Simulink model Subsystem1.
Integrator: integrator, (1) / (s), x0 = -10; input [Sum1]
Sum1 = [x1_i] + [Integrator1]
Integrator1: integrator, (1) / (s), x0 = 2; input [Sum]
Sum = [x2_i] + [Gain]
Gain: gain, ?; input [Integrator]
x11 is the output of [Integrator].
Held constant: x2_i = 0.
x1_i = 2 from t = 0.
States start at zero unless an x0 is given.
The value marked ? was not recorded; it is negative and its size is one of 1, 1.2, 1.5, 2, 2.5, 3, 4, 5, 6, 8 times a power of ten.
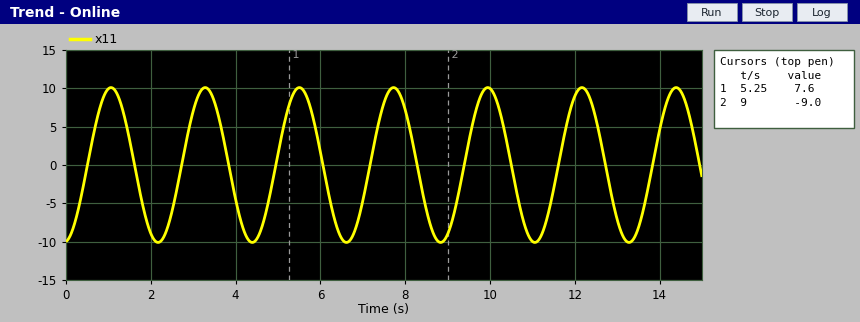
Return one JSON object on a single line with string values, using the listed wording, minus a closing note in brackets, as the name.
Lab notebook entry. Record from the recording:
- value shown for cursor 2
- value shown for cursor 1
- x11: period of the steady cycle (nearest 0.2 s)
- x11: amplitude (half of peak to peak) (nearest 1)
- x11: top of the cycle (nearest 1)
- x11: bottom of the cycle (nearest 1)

{"value shown for cursor 2": "-9.0", "value shown for cursor 1": "7.6", "x11: period of the steady cycle": "2.2 s", "x11: amplitude (half of peak to peak)": "10", "x11: top of the cycle": "10", "x11: bottom of the cycle": "-10"}
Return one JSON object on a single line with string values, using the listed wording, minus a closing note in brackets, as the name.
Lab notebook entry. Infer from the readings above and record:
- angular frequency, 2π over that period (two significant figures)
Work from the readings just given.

{"angular frequency, 2π over that period": "2.9 rad/s"}
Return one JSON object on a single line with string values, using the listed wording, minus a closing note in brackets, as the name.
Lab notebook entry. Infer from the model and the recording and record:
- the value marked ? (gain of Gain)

{"the value marked ?": "-8"}
